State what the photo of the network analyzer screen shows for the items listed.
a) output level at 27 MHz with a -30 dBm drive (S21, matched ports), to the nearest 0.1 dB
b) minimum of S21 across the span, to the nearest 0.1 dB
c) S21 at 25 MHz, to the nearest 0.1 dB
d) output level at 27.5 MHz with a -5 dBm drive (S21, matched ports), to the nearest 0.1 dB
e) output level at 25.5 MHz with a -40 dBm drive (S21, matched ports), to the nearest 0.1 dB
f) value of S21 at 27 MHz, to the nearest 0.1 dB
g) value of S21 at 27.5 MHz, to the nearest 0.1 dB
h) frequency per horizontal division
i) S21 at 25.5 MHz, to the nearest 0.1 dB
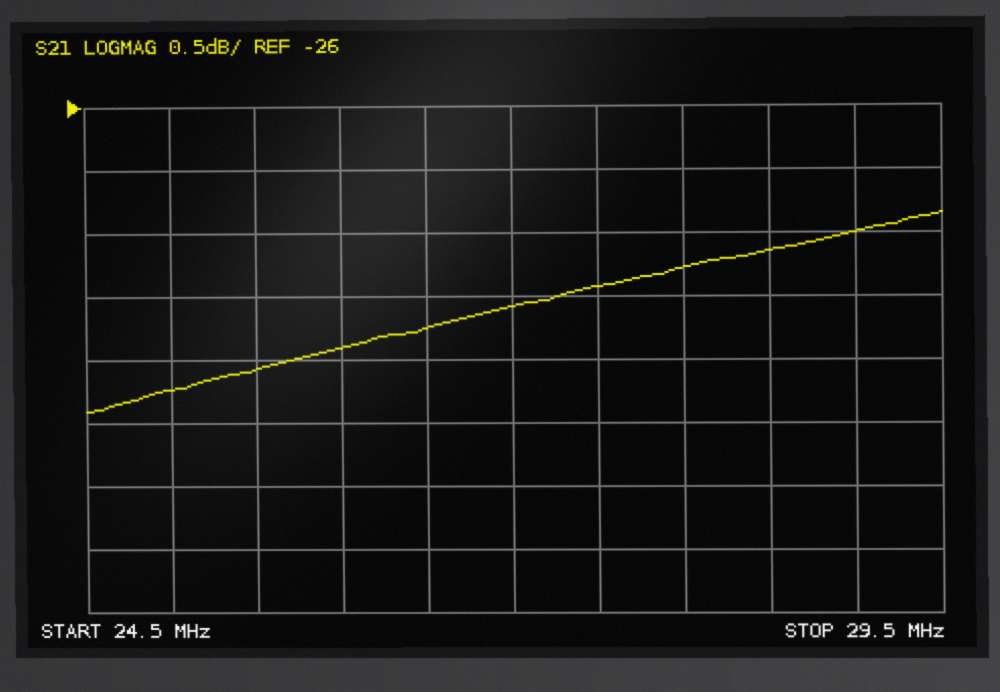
-57.6 dBm
-28.4 dB
-28.2 dB
-32.4 dBm
-68.1 dBm
-27.6 dB
-27.4 dB
500 kHz
-28.1 dB
